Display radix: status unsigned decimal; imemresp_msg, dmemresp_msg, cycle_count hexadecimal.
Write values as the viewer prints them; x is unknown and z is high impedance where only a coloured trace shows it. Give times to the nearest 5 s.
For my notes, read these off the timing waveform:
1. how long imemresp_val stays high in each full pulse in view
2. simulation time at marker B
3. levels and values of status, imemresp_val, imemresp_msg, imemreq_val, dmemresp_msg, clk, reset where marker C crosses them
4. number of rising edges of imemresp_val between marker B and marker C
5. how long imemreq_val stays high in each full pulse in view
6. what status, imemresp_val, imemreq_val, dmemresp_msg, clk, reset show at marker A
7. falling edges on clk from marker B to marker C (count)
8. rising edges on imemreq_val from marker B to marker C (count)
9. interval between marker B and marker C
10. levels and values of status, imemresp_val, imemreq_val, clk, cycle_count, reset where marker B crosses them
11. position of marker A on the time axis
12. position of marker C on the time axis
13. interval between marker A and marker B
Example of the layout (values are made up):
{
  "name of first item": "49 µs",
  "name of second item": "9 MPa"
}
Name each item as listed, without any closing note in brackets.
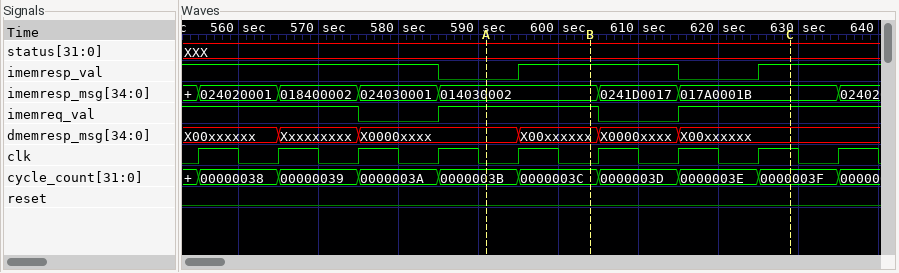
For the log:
{
  "how long imemresp_val stays high in each full pulse in view": "20 s",
  "simulation time at marker B": "605 s",
  "levels and values of status, imemresp_val, imemresp_msg, imemreq_val, dmemresp_msg, clk, reset where marker C crosses them": "status=XXX, imemresp_val=1, imemresp_msg=017A0001B, imemreq_val=1, dmemresp_msg=X00xxxxxx, clk=1, reset=0",
  "number of rising edges of imemresp_val between marker B and marker C": "1",
  "how long imemreq_val stays high in each full pulse in view": "20 s",
  "what status, imemresp_val, imemreq_val, dmemresp_msg, clk, reset show at marker A": "status=XXX, imemresp_val=0, imemreq_val=1, dmemresp_msg=X0000xxxx, clk=0, reset=0",
  "falling edges on clk from marker B to marker C": "2",
  "rising edges on imemreq_val from marker B to marker C": "1",
  "interval between marker B and marker C": "25 s",
  "levels and values of status, imemresp_val, imemreq_val, clk, cycle_count, reset where marker B crosses them": "status=XXX, imemresp_val=1, imemreq_val=1, clk=0, cycle_count=0000003C, reset=0",
  "position of marker A on the time axis": "590 s",
  "position of marker C on the time axis": "630 s",
  "interval between marker A and marker B": "15 s"
}
